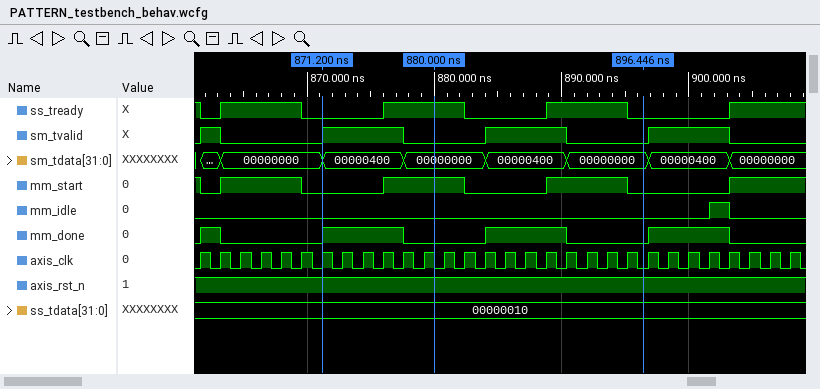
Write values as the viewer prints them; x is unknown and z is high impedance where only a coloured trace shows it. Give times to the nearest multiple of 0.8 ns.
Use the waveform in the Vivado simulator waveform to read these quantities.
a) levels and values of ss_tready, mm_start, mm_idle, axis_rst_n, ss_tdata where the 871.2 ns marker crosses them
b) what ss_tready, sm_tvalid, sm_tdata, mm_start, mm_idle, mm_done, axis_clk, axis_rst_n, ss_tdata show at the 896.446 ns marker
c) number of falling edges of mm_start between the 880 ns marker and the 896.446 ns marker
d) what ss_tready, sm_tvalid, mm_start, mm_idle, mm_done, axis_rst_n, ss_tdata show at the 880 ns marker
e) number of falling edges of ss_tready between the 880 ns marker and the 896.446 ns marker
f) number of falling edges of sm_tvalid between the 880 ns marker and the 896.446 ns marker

ss_tready=0, mm_start=0, mm_idle=0, axis_rst_n=1, ss_tdata=00000010
ss_tready=0, sm_tvalid=0, sm_tdata=00000000, mm_start=0, mm_idle=0, mm_done=0, axis_clk=0, axis_rst_n=1, ss_tdata=00000010
2
ss_tready=1, sm_tvalid=0, mm_start=1, mm_idle=0, mm_done=0, axis_rst_n=1, ss_tdata=00000010
2
1
